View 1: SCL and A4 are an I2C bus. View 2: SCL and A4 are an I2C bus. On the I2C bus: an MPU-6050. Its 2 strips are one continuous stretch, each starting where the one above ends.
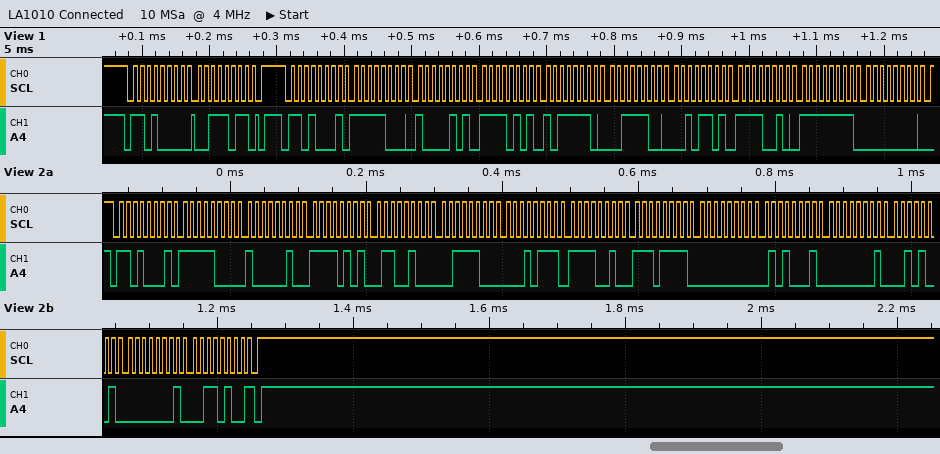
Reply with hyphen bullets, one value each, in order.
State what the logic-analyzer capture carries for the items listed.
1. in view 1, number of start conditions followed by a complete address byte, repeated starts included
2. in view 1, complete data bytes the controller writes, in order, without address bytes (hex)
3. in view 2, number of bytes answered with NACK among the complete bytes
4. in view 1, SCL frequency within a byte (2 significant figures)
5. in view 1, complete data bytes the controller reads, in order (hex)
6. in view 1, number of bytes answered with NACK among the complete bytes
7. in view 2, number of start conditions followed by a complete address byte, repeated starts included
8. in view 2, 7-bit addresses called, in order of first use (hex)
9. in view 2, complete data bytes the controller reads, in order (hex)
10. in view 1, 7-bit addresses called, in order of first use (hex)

- 2
- 3B
- 1
- 100 kHz
- F8 85 F5 BE 3C 2D F2 FF 00
- 0
- 1
- 0x68
- F8 82 F5 64 3C 17 F2 EF 00 51 01 29 01 34
- 0x68
